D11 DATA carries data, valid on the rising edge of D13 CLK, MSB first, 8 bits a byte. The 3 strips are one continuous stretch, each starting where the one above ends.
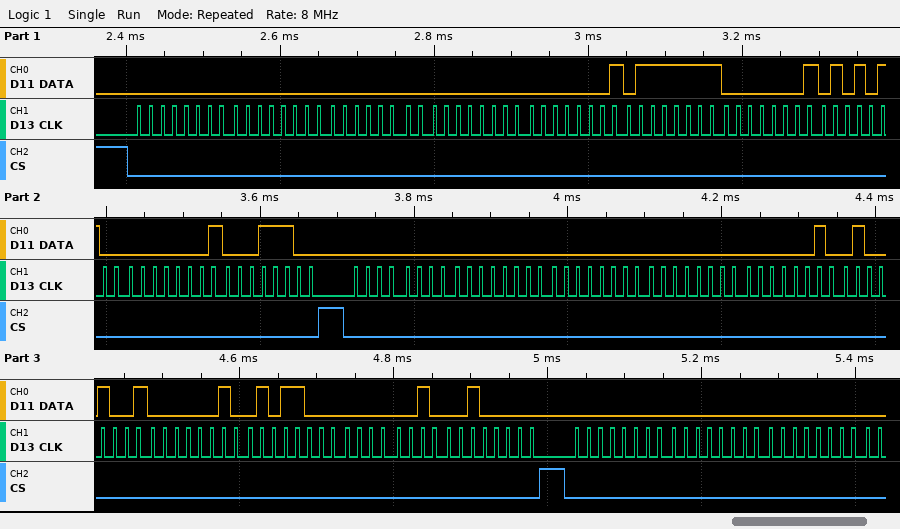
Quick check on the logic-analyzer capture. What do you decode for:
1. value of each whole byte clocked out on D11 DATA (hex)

00 00 00 00 01 7F 01 54 01 1C 00 00 00 00 02 49 02 58 02 20 00 00 00
